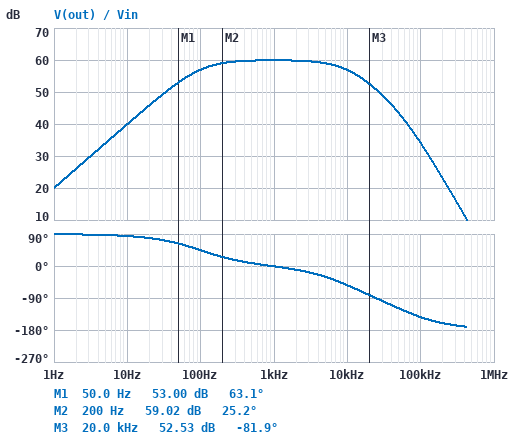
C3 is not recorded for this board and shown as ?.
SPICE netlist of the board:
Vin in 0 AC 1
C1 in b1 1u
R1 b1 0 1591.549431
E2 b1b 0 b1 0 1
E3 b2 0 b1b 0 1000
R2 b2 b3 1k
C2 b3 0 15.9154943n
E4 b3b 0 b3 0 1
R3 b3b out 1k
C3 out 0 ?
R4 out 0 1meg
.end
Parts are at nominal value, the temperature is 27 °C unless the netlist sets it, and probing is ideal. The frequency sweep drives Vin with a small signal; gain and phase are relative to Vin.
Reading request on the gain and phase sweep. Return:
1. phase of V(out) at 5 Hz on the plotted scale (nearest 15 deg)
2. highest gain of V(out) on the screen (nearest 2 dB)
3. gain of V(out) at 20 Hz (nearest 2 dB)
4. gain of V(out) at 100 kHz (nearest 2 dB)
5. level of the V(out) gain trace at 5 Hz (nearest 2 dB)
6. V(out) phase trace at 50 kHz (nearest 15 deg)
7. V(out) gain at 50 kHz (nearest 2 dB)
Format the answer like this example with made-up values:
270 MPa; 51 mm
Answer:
90 deg; 60 dB; 46 dB; 34 dB; 34 dB; -120 deg; 44 dB
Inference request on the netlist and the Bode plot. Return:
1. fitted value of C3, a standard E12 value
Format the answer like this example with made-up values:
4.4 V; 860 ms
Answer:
2.7 nF
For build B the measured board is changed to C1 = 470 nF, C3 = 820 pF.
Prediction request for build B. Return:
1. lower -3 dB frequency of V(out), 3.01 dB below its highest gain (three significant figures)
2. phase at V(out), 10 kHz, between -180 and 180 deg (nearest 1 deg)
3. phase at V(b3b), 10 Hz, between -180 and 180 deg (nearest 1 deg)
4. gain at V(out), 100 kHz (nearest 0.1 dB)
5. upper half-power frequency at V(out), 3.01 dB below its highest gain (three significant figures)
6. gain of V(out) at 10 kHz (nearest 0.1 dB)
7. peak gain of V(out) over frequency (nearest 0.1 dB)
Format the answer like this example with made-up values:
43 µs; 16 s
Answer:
204 Hz; -47 deg; 87 deg; 38.9 dB; 10.4 kHz; 57.0 dB; 59.8 dB
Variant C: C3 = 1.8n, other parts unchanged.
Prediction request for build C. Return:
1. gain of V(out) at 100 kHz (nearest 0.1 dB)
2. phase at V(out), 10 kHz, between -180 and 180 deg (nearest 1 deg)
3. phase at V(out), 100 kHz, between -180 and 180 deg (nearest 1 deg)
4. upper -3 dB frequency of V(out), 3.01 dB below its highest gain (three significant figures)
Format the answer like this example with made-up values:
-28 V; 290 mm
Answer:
36.4 dB; -51 deg; -133 deg; 10.1 kHz
